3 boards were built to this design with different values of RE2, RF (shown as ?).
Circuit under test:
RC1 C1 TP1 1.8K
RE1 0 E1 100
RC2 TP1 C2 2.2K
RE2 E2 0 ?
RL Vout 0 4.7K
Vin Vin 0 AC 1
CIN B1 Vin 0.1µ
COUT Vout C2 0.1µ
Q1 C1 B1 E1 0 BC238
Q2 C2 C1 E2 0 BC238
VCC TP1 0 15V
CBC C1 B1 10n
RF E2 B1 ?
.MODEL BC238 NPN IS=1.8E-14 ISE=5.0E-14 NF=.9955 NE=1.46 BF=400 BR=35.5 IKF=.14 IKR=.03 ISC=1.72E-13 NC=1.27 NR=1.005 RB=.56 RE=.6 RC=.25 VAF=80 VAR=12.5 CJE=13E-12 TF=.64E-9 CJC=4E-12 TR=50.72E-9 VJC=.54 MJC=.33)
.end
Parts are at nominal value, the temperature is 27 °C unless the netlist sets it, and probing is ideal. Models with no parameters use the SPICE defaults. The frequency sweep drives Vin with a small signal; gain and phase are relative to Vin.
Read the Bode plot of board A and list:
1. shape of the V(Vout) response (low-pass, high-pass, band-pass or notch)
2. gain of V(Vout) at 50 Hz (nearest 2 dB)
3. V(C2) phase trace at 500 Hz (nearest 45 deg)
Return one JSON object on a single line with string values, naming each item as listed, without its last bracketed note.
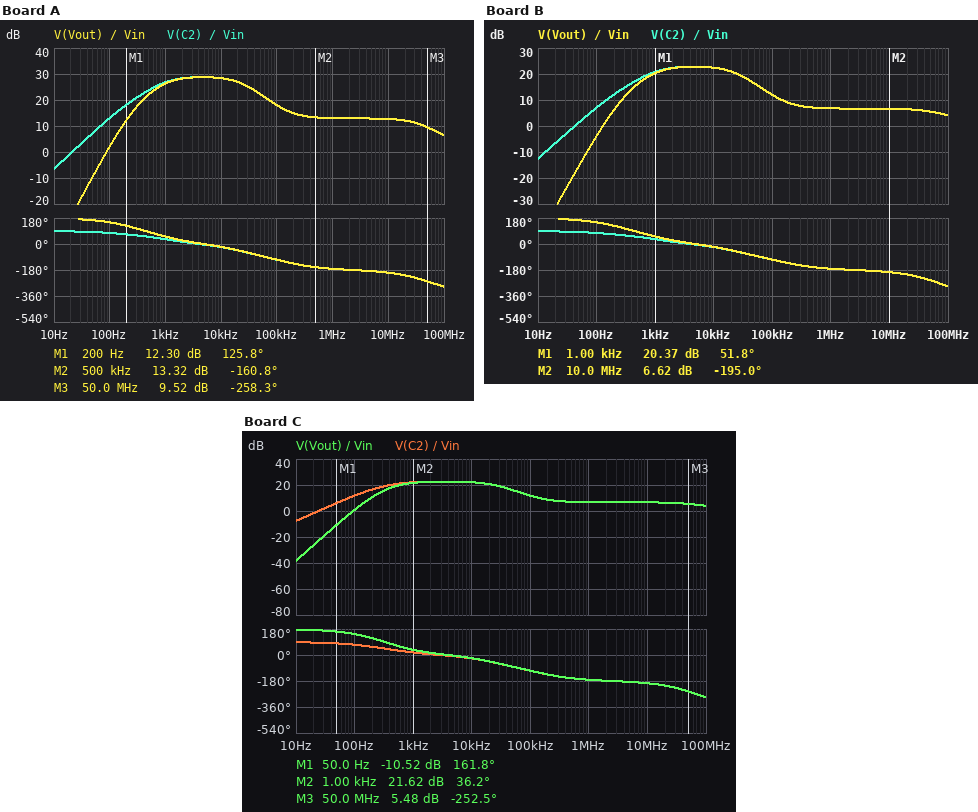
{"shape of the V(Vout) response": "band-pass", "gain of V(Vout) at 50 Hz": "-10 dB", "V(C2) phase trace at 500 Hz": "45 deg"}
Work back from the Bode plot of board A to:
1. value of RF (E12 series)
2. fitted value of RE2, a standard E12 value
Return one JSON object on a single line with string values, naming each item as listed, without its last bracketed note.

{"value of RF": "12 kΩ", "fitted value of RE2, a standard E12 value": "330 Ω"}
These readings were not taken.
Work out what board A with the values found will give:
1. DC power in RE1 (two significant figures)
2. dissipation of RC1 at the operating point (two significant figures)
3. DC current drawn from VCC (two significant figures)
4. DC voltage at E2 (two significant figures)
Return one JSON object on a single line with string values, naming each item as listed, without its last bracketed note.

{"DC power in RE1": "4.9 mW", "dissipation of RC1 at the operating point": "89 mW", "DC current drawn from VCC": "12 mA", "DC voltage at E2": "1.7 V"}
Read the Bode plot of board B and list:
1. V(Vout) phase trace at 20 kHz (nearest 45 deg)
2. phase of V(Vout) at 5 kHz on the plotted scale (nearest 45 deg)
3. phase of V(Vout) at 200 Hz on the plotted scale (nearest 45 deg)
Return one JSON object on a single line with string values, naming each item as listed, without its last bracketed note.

{"V(Vout) phase trace at 20 kHz": "-45 deg", "phase of V(Vout) at 5 kHz on the plotted scale": "0 deg", "phase of V(Vout) at 200 Hz on the plotted scale": "135 deg"}
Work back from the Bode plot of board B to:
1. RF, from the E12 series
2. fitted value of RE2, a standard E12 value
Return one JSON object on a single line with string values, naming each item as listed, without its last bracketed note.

{"RF, from the E12 series": "12 kΩ", "fitted value of RE2, a standard E12 value": "680 Ω"}
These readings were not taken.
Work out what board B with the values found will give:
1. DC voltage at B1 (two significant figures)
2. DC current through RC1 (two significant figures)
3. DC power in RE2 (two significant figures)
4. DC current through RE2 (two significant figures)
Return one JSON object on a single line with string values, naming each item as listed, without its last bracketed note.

{"DC voltage at B1": "1.4 V", "DC current through RC1": "7.0 mA", "DC power in RE2": "4.2 mW", "DC current through RE2": "2.5 mA"}
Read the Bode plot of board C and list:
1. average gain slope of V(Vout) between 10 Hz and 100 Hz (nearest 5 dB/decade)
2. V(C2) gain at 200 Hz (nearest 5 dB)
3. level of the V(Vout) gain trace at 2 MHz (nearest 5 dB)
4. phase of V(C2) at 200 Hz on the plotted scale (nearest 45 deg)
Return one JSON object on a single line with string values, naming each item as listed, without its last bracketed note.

{"average gain slope of V(Vout) between 10 Hz and 100 Hz": "40 dB/decade", "V(C2) gain at 200 Hz": "15 dB", "level of the V(Vout) gain trace at 2 MHz": "5 dB", "phase of V(C2) at 200 Hz on the plotted scale": "45 deg"}
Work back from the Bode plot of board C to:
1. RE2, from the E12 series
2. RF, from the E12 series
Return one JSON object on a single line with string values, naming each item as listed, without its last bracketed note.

{"RE2, from the E12 series": "680 Ω", "RF, from the E12 series": "22 kΩ"}
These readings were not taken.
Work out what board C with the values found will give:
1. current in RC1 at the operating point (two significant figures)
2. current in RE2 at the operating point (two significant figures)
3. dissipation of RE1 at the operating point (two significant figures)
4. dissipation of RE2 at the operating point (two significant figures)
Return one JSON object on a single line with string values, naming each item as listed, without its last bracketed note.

{"current in RC1 at the operating point": "6.9 mA", "current in RE2 at the operating point": "2.8 mA", "dissipation of RE1 at the operating point": "4.8 mW", "dissipation of RE2 at the operating point": "5.3 mW"}
